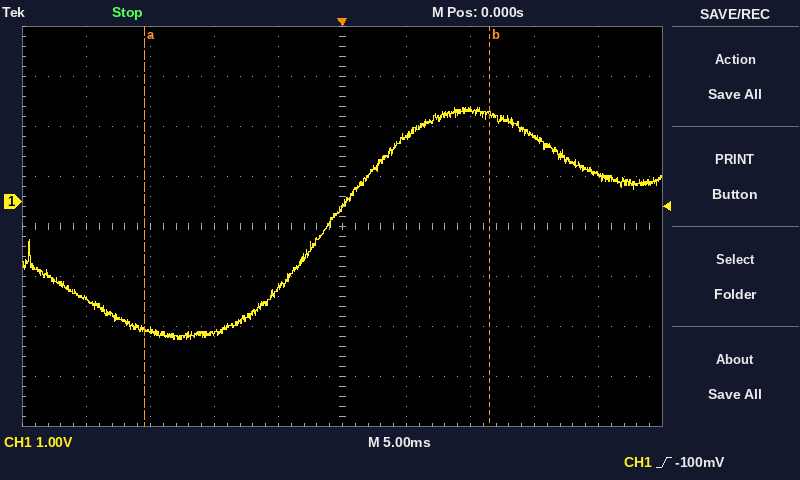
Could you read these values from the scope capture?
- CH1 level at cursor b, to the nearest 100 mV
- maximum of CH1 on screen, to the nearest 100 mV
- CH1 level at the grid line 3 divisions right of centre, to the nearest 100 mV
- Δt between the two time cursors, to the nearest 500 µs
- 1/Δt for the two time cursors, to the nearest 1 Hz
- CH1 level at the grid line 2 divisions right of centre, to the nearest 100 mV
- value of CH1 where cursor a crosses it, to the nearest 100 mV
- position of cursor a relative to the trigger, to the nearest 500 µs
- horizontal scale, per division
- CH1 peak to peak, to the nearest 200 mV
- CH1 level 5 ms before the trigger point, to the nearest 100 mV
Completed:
1.7 V
1.9 V
1.3 V
27.0 ms
37 Hz
1.8 V
-2.5 V
-15.5 ms
5 ms
4.6 V
-1.7 V
